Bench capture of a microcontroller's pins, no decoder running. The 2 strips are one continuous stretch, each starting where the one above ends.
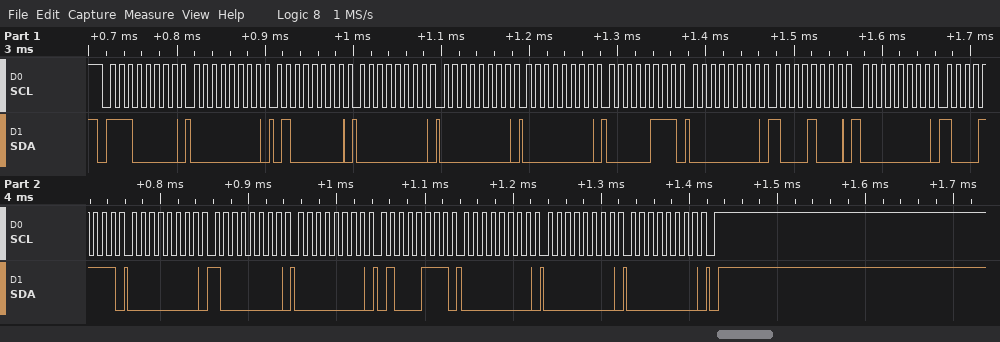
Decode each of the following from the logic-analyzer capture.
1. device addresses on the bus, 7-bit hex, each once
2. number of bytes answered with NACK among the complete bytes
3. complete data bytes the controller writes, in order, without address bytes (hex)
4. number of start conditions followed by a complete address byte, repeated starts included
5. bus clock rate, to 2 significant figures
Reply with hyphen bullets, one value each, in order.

- 0x70
- 0
- 00 40 00 00 00 07 00 88 00 8F 00 80 00 47 00 00 00
- 1
- 100 kHz
